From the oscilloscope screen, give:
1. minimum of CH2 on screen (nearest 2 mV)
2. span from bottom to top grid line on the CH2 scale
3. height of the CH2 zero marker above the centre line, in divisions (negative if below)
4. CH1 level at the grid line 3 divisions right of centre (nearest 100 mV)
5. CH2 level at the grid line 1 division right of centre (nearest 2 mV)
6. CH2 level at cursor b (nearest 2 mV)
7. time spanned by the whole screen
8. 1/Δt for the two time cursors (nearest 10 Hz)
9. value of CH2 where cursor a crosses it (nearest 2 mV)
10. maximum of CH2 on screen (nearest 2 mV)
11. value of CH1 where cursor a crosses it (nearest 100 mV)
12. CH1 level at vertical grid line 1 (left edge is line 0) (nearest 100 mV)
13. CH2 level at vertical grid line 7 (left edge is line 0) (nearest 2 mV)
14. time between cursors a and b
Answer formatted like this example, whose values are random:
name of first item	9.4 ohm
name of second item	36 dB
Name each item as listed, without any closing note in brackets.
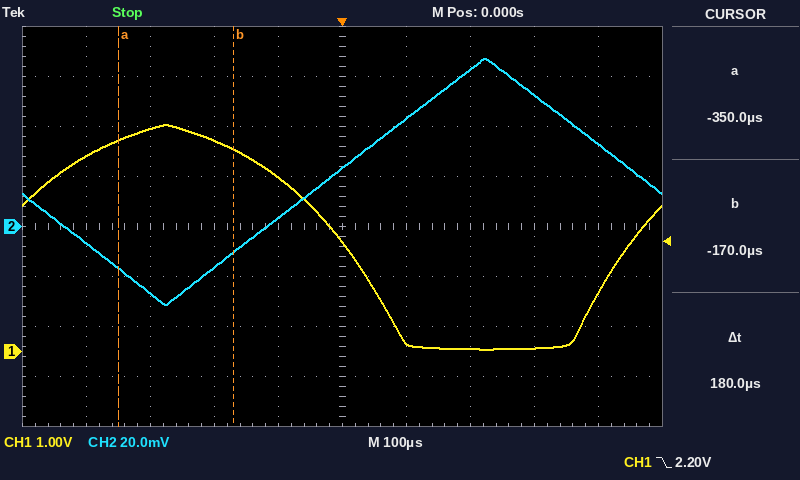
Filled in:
minimum of CH2 on screen	-32 mV
span from bottom to top grid line on the CH2 scale	160 mV
height of the CH2 zero marker above the centre line, in divisions	0.0 div
CH1 level at the grid line 3 divisions right of centre	100 mV
CH2 level at the grid line 1 division right of centre	44 mV
CH2 level at cursor b	-10 mV
time spanned by the whole screen	1 ms
1/Δt for the two time cursors	5.56 kHz
value of CH2 where cursor a crosses it	-16 mV
maximum of CH2 on screen	68 mV
value of CH1 where cursor a crosses it	4.2 V
CH1 level at vertical grid line 1 (left edge is line 0)	3.9 V
CH2 level at vertical grid line 7 (left edge is line 0)	62 mV
time between cursors a and b	180 µs
